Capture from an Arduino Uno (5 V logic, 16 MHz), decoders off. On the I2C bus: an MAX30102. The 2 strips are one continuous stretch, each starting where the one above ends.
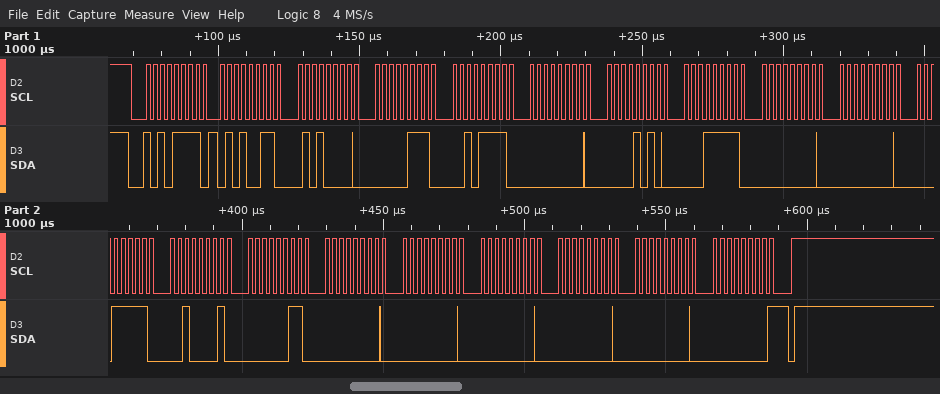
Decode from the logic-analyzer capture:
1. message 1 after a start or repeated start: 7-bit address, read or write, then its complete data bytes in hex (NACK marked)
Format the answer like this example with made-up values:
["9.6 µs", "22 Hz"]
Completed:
["0x57 read: 53 50 07 2F 00 0A 1F 00 00 1F 21 03 00 00 00 00 00 00 NACK"]
